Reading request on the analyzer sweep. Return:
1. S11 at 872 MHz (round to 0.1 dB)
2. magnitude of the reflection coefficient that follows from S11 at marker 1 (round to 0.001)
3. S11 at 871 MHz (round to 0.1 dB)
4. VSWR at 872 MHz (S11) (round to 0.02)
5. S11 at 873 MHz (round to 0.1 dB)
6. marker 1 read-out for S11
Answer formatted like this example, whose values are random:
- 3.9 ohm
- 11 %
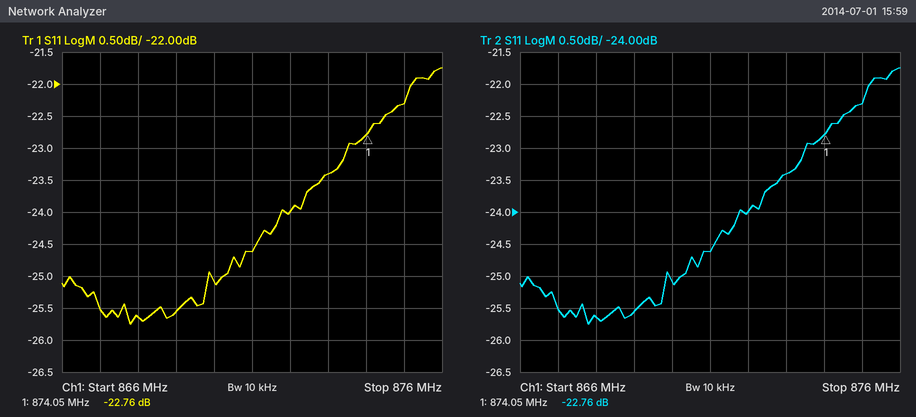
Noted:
- -24.0 dB
- 0.073
- -24.6 dB
- 1.14
- -23.4 dB
- -22.76 dB
